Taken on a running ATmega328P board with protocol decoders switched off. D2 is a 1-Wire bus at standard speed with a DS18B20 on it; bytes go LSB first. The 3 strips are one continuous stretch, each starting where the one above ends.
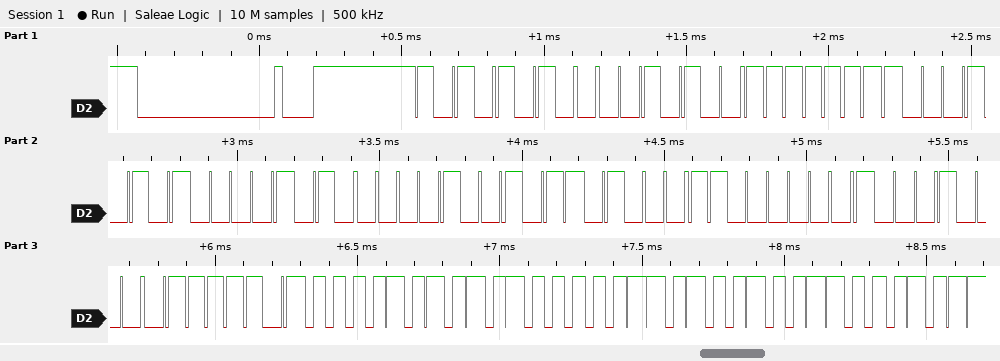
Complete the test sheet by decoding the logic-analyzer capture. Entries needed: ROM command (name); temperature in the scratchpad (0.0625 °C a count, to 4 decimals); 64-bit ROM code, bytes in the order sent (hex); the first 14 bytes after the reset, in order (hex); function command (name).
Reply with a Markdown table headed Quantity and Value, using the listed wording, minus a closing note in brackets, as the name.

| Quantity | Value |
|---|---|
| ROM command | Match ROM |
| temperature in the scratchpad | 85.0000 °C |
| 64-bit ROM code, bytes in the order sent | 28 FF A8 50 90 16 03 11 |
| the first 14 bytes after the reset, in order | 55 28 FF A8 50 90 16 03 11 BE 50 05 4B 46 |
| function command | Read Scratchpad |
